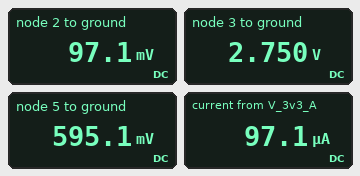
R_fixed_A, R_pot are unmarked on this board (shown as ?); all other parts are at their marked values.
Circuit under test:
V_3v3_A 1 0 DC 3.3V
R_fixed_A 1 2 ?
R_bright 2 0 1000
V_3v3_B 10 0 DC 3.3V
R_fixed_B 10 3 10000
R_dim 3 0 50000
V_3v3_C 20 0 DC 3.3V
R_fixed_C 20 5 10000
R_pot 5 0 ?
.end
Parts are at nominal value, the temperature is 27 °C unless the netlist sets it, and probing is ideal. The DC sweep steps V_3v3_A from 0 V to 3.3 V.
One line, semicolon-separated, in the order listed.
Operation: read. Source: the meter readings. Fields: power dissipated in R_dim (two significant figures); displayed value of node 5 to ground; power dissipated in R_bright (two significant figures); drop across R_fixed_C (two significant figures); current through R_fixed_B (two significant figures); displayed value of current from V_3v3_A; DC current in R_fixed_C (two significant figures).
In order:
150 µW; 595.1 mV; 9.4 µW; 2.7 V; 55 µA; 97.1 µA; 270 µA
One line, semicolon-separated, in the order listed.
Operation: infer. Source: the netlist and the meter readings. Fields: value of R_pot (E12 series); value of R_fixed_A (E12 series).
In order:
2.2 kΩ; 33 kΩ
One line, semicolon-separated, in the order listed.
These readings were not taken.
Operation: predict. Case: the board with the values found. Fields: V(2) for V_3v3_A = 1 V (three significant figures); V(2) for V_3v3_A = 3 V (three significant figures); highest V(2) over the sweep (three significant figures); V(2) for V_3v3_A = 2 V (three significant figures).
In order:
29.4 mV; 88.2 mV; 97.1 mV; 58.8 mV
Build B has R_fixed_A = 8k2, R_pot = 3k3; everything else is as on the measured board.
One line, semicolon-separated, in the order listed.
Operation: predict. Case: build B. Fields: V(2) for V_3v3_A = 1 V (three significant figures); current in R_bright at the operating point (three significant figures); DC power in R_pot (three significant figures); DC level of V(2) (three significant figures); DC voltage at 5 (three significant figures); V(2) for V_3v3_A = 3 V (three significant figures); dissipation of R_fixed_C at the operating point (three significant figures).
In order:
109 mV; 359 µA; 203 µW; 359 mV; 819 mV; 326 mV; 616 µW
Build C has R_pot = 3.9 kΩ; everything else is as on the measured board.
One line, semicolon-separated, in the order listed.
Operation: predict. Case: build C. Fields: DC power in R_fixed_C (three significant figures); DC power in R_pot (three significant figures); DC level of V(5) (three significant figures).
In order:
564 µW; 220 µW; 926 mV
